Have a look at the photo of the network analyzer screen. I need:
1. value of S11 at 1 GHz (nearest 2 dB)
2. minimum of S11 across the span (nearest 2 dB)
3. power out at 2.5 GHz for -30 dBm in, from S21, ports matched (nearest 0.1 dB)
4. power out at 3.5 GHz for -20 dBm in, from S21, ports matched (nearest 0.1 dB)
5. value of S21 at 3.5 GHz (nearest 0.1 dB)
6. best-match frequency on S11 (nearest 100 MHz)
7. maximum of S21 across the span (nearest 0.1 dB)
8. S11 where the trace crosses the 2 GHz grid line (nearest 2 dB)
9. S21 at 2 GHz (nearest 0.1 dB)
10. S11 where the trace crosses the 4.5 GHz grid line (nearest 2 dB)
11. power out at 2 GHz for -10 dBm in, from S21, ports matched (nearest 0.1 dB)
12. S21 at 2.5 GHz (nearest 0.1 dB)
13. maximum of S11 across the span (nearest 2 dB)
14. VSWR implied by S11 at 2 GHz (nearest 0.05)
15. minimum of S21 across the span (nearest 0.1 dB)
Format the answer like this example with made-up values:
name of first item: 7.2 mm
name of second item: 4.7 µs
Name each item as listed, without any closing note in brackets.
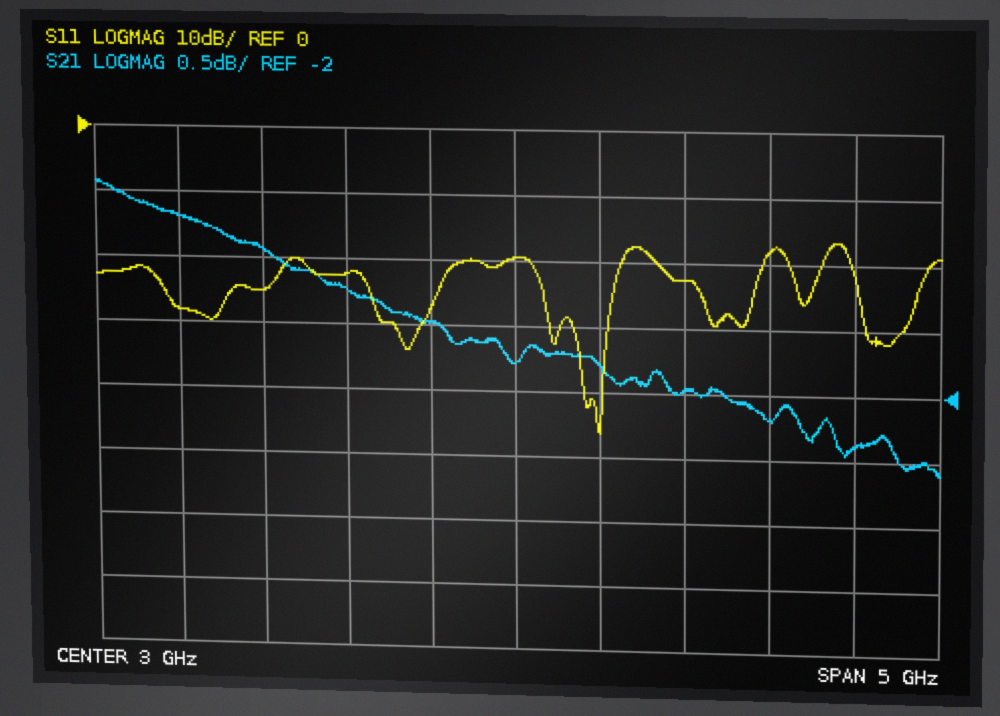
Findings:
value of S11 at 1 GHz: -28 dB
minimum of S11 across the span: -46 dB
power out at 2.5 GHz for -30 dBm in, from S21, ports matched: -31.5 dBm
power out at 3.5 GHz for -20 dBm in, from S21, ports matched: -21.8 dBm
value of S21 at 3.5 GHz: -1.8 dB
best-match frequency on S11: 3.5 GHz
maximum of S21 across the span: -0.4 dB
S11 where the trace crosses the 2 GHz grid line: -22 dB
S21 at 2 GHz: -1.2 dB
S11 where the trace crosses the 4.5 GHz grid line: -18 dB
power out at 2 GHz for -10 dBm in, from S21, ports matched: -11.2 dBm
S21 at 2.5 GHz: -1.5 dB
maximum of S11 across the span: -16 dB
VSWR implied by S11 at 2 GHz: 1.15
minimum of S21 across the span: -2.6 dB
